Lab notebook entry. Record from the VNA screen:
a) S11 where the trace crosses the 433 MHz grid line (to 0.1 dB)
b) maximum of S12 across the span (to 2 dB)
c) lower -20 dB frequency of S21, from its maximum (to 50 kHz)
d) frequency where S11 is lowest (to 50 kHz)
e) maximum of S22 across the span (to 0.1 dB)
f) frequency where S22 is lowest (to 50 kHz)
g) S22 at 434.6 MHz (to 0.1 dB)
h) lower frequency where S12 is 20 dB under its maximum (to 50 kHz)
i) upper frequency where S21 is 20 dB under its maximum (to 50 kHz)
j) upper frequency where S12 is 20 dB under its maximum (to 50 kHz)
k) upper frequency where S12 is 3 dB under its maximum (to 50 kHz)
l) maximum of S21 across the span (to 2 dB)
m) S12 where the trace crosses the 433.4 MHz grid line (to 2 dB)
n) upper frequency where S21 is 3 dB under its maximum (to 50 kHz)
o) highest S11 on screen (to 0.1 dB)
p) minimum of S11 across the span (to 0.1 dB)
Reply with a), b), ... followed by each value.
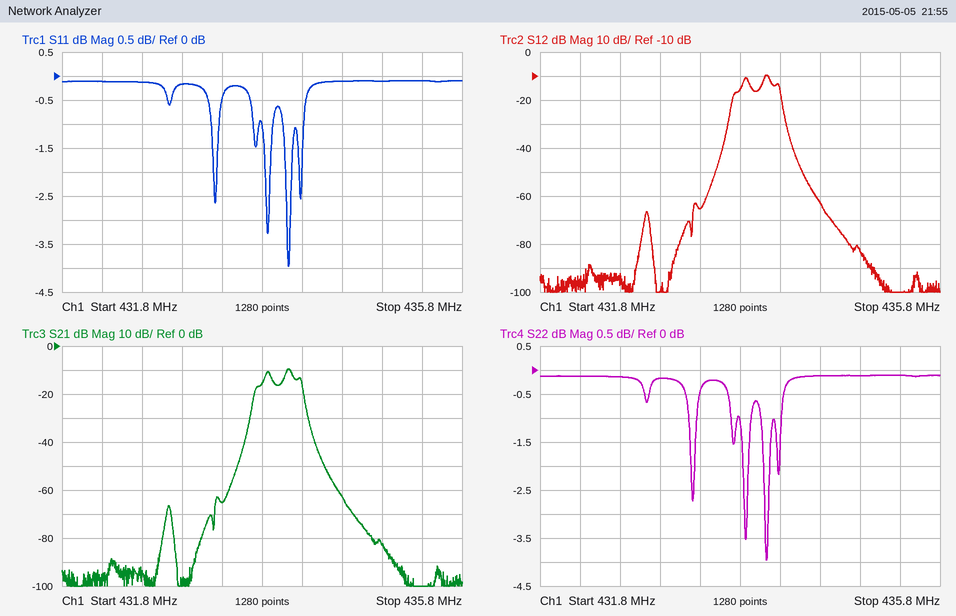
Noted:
a) -0.2 dB
b) -10 dB
c) 433.70 MHz
d) 434.05 MHz
e) -0.1 dB
f) 434.05 MHz
g) -0.1 dB
h) 433.70 MHz
i) 434.25 MHz
j) 434.25 MHz
k) 434.10 MHz
l) -10 dB
m) -66 dB
n) 434.10 MHz
o) -0.1 dB
p) -4.0 dB
